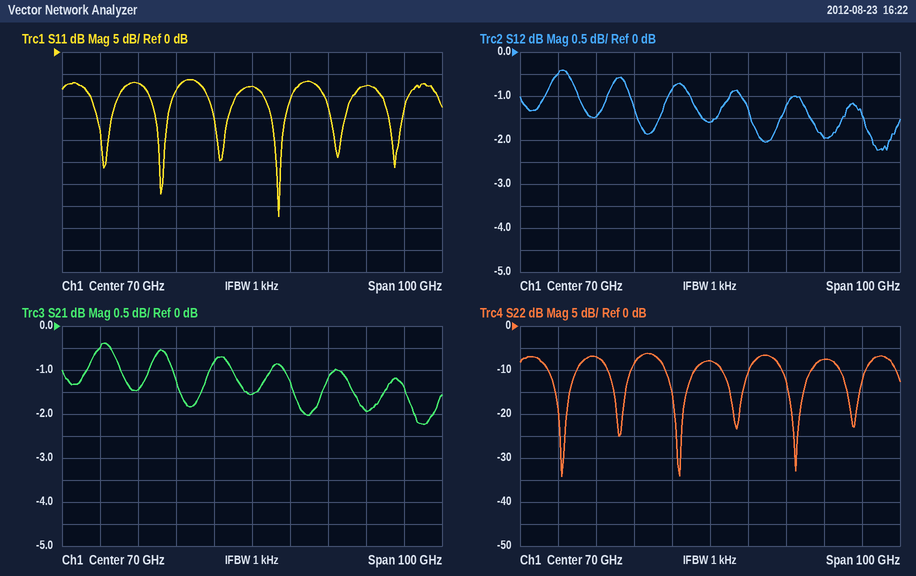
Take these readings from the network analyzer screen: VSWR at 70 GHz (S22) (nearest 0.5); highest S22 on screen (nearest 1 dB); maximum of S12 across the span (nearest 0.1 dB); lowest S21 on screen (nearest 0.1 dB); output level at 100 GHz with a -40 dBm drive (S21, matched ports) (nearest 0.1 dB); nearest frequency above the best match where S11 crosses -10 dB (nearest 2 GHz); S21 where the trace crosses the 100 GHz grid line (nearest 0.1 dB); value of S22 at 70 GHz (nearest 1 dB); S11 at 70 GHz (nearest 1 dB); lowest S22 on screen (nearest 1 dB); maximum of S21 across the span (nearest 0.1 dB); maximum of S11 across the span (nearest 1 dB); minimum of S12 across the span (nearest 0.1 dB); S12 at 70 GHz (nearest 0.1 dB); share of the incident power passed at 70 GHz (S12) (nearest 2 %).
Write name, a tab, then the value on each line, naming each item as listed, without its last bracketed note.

VSWR at 70 GHz (S22)	2.5
highest S22 on screen	-6 dB
maximum of S12 across the span	-0.4 dB
lowest S21 on screen	-2.2 dB
output level at 100 GHz with a -40 dBm drive (S21, matched ports)	-41.9 dBm
nearest frequency above the best match where S11 crosses -10 dB	80 GHz
S21 where the trace crosses the 100 GHz grid line	-1.9 dB
value of S22 at 70 GHz	-8 dB
S11 at 70 GHz	-8 dB
lowest S22 on screen	-34 dB
maximum of S21 across the span	-0.4 dB
maximum of S11 across the span	-6 dB
minimum of S12 across the span	-2.2 dB
S12 at 70 GHz	-1.6 dB
share of the incident power passed at 70 GHz (S12)	70 %
